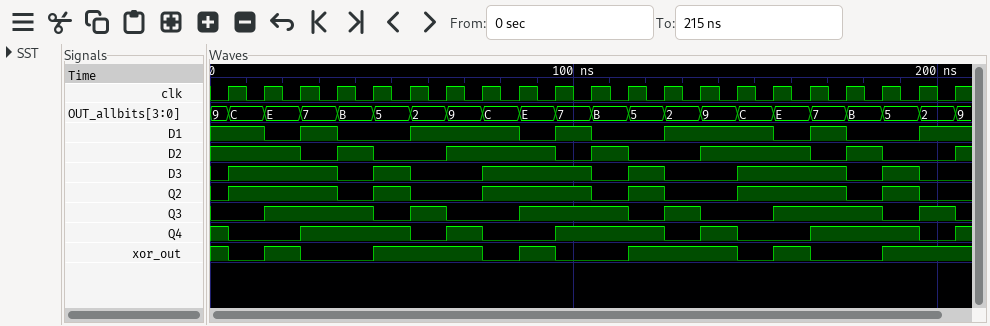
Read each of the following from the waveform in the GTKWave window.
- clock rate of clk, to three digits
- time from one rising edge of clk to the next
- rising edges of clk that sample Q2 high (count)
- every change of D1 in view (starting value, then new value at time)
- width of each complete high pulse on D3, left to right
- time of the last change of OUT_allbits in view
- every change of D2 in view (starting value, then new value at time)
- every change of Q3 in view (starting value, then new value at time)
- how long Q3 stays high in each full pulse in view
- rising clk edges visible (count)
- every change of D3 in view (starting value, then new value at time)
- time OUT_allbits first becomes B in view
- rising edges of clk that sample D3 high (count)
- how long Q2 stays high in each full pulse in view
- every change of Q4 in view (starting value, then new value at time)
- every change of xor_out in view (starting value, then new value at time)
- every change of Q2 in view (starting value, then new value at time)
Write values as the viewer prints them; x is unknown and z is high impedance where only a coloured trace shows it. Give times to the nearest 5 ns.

100 MHz
10 ns
12
1, 0 at 15 ns, 1 at 25 ns, 0 at 35 ns, 1 at 55 ns, 0 at 85 ns, 1 at 95 ns, 0 at 105 ns, 1 at 125 ns, 0 at 155 ns, 1 at 165 ns, 0 at 175 ns, 1 at 195 ns
30 ns, 10 ns, 30 ns, 10 ns, 30 ns, 10 ns
205 ns
1, 0 at 25 ns, 1 at 35 ns, 0 at 45 ns, 1 at 65 ns, 0 at 95 ns, 1 at 105 ns, 0 at 115 ns, 1 at 135 ns, 0 at 165 ns, 1 at 175 ns, 0 at 185 ns, 1 at 205 ns
0, 1 at 15 ns, 0 at 45 ns, 1 at 55 ns, 0 at 65 ns, 1 at 85 ns, 0 at 115 ns, 1 at 125 ns, 0 at 135 ns, 1 at 155 ns, 0 at 185 ns, 1 at 195 ns, 0 at 205 ns
30 ns, 10 ns, 30 ns, 10 ns, 30 ns, 10 ns
21
0, 1 at 5 ns, 0 at 35 ns, 1 at 45 ns, 0 at 55 ns, 1 at 75 ns, 0 at 105 ns, 1 at 115 ns, 0 at 125 ns, 1 at 145 ns, 0 at 175 ns, 1 at 185 ns, 0 at 195 ns
35 ns
12
30 ns, 10 ns, 30 ns, 10 ns, 30 ns, 10 ns
1, 0 at 5 ns, 1 at 25 ns, 0 at 55 ns, 1 at 65 ns, 0 at 75 ns, 1 at 95 ns, 0 at 125 ns, 1 at 135 ns, 0 at 145 ns, 1 at 165 ns, 0 at 195 ns, 1 at 205 ns
1, 0 at 5 ns, 1 at 15 ns, 0 at 25 ns, 1 at 45 ns, 0 at 75 ns, 1 at 85 ns, 0 at 95 ns, 1 at 115 ns, 0 at 145 ns, 1 at 155 ns, 0 at 165 ns, 1 at 185 ns
0, 1 at 5 ns, 0 at 35 ns, 1 at 45 ns, 0 at 55 ns, 1 at 75 ns, 0 at 105 ns, 1 at 115 ns, 0 at 125 ns, 1 at 145 ns, 0 at 175 ns, 1 at 185 ns, 0 at 195 ns
